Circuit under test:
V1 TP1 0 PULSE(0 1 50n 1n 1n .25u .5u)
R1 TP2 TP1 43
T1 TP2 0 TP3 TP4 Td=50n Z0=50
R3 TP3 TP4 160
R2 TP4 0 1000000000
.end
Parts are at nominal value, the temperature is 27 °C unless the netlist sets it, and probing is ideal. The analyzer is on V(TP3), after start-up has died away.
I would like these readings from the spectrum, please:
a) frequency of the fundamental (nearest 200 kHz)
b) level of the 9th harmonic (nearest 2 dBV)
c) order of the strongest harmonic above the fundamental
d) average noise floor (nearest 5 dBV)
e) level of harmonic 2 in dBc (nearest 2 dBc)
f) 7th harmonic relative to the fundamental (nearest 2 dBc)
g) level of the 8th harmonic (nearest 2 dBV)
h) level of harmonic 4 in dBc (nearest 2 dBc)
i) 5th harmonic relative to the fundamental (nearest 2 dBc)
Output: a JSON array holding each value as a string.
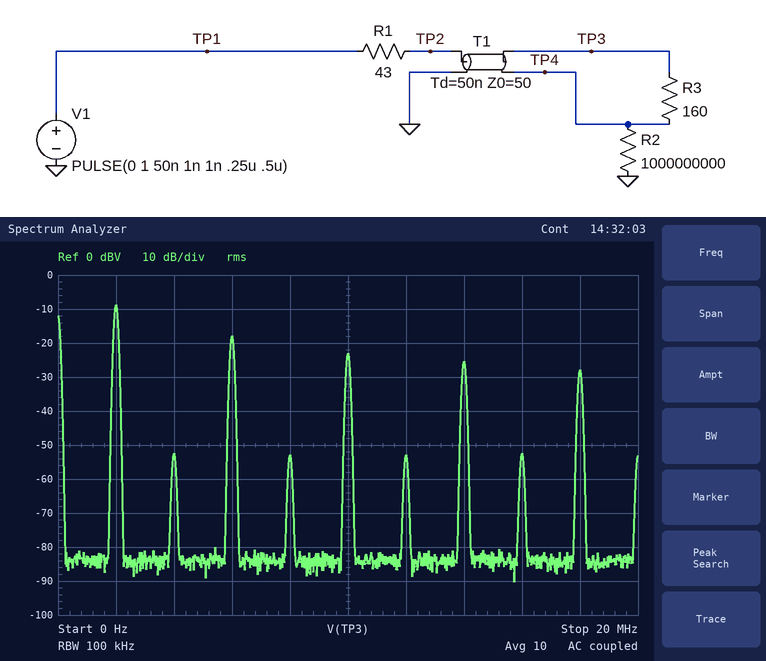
["2.0 MHz", "-28 dBV", "3", "-85 dBV", "-44 dBc", "-16 dBc", "-52 dBV", "-44 dBc", "-14 dBc"]
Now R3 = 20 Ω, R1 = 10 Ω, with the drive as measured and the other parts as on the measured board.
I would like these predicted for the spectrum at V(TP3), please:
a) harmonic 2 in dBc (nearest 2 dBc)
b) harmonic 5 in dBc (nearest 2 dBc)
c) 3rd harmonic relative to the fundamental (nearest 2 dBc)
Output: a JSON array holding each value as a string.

["-46 dBc", "-12 dBc", "-12 dBc"]
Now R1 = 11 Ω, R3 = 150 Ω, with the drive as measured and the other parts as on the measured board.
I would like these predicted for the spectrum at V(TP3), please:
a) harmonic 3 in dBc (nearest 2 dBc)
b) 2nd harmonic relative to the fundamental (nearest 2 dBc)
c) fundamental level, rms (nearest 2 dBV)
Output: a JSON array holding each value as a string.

["-6 dBc", "-40 dBc", "-6 dBV"]
